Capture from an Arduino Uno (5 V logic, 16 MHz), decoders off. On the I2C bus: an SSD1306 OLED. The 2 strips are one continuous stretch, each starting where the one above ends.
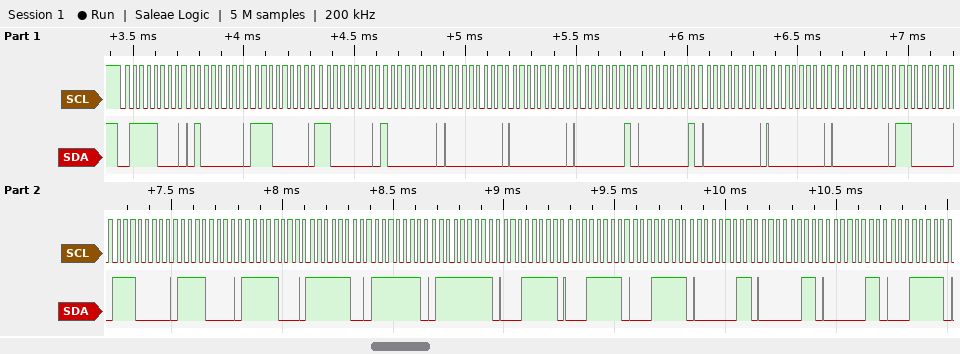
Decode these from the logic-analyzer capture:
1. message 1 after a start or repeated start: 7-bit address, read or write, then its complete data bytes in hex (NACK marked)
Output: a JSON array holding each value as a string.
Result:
["0x3C write: 40 E0 C0 80 00 00 01 01 00 00 00 C0 E0 F0 F8 FC FE FF 1F 1F 1F 03 03 03 1F"]
